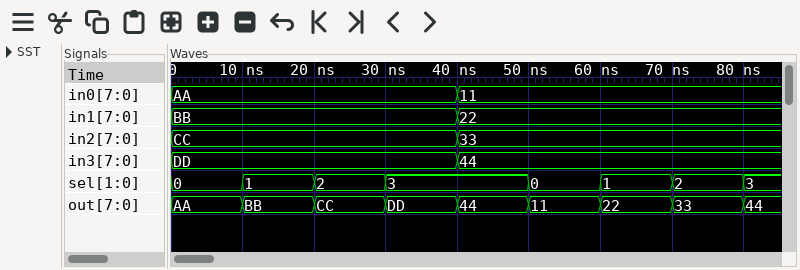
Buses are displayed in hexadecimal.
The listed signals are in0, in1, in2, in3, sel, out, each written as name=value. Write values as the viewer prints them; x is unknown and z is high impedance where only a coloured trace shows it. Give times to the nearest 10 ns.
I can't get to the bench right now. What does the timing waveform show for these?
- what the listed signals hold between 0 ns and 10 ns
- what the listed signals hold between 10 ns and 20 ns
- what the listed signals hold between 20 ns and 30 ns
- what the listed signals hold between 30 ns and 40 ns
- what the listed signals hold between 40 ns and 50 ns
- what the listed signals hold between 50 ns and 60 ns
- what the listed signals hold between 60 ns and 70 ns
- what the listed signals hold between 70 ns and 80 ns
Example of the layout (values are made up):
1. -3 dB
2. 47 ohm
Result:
1. in0=AA, in1=BB, in2=CC, in3=DD, sel=0, out=AA
2. in0=AA, in1=BB, in2=CC, in3=DD, sel=1, out=BB
3. in0=AA, in1=BB, in2=CC, in3=DD, sel=2, out=CC
4. in0=AA, in1=BB, in2=CC, in3=DD, sel=3, out=DD
5. in0=11, in1=22, in2=33, in3=44, sel=3, out=44
6. in0=11, in1=22, in2=33, in3=44, sel=0, out=11
7. in0=11, in1=22, in2=33, in3=44, sel=1, out=22
8. in0=11, in1=22, in2=33, in3=44, sel=2, out=33
